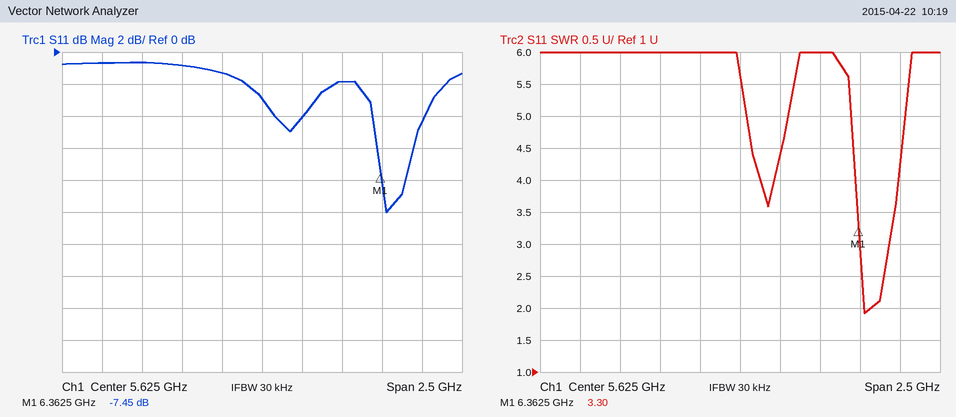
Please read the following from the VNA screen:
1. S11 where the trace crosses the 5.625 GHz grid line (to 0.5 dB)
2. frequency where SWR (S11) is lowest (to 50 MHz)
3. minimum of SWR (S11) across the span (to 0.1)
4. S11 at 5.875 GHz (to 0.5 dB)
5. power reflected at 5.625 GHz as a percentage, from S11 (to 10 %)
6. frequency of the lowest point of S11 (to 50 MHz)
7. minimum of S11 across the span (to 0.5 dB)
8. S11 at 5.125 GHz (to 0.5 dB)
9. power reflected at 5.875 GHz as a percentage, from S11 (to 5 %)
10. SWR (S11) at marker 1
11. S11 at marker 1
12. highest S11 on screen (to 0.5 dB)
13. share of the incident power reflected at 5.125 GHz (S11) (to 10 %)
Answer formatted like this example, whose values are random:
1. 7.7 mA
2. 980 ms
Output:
1. -3.0 dB
2. 6.40 GHz
3. 1.9
4. -4.0 dB
5. 50 %
6. 6.40 GHz
7. -10.0 dB
8. -1.0 dB
9. 40 %
10. 3.30
11. -7.45 dB
12. -0.5 dB
13. 80 %
